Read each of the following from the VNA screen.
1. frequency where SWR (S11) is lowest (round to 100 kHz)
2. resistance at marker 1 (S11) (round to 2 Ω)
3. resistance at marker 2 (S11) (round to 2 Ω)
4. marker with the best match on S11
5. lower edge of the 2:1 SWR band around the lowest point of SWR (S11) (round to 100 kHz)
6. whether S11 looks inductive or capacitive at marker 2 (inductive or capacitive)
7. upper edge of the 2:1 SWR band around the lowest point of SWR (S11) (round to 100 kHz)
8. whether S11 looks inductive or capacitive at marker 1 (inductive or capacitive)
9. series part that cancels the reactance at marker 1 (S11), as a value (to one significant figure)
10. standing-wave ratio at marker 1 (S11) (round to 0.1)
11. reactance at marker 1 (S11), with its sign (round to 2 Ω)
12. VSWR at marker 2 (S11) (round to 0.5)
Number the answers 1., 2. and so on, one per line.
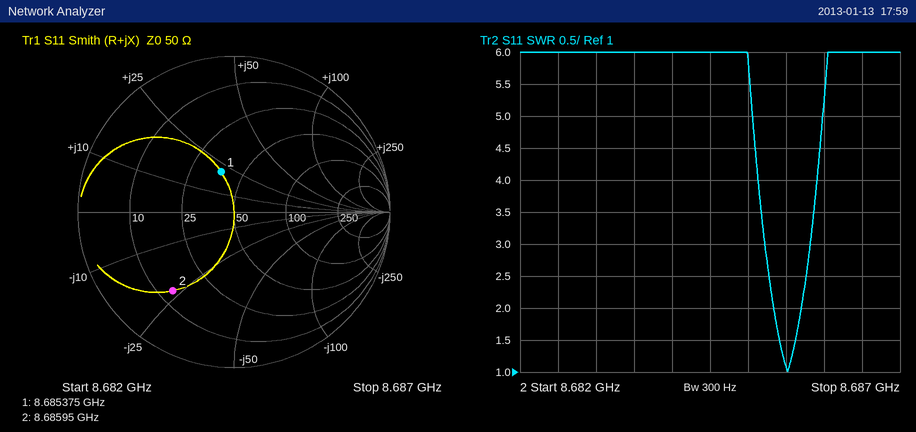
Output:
1. 8.6855 GHz
2. 38 Ω
3. 14 Ω
4. marker 1
5. 8.6853 GHz
6. capacitive
7. 8.6857 GHz
8. inductive
9. 900 fF
10. 1.7
11. +20 Ω
12. 4.5
